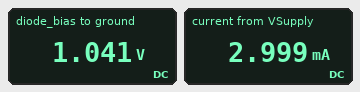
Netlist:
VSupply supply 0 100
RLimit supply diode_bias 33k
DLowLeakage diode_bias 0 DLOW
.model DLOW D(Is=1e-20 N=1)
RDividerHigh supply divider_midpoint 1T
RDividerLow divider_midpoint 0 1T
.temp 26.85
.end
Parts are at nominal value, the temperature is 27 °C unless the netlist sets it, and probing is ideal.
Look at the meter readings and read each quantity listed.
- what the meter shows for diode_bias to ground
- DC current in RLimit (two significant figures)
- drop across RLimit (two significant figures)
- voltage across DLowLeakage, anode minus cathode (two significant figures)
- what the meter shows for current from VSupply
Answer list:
1.041 V
3.0 mA
99 V
1.0 V
2.999 mA
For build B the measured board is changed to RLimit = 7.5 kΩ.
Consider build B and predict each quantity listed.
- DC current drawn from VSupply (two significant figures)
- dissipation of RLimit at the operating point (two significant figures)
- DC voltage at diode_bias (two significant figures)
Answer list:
13 mA
1.3 W
1.1 V
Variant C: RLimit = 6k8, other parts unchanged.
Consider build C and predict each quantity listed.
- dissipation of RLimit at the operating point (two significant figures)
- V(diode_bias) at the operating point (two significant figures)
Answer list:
1.4 W
1.1 V
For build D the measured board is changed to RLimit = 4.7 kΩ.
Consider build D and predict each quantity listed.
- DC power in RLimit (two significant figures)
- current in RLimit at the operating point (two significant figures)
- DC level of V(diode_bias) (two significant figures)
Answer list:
2.1 W
21 mA
1.1 V
